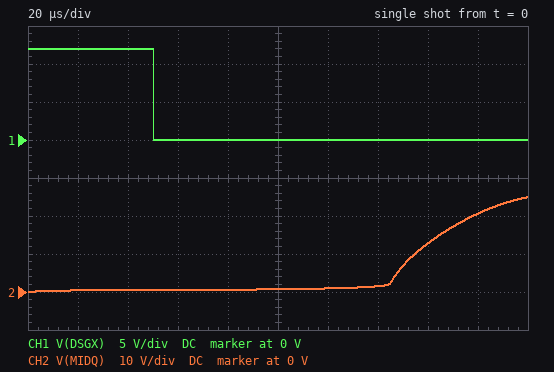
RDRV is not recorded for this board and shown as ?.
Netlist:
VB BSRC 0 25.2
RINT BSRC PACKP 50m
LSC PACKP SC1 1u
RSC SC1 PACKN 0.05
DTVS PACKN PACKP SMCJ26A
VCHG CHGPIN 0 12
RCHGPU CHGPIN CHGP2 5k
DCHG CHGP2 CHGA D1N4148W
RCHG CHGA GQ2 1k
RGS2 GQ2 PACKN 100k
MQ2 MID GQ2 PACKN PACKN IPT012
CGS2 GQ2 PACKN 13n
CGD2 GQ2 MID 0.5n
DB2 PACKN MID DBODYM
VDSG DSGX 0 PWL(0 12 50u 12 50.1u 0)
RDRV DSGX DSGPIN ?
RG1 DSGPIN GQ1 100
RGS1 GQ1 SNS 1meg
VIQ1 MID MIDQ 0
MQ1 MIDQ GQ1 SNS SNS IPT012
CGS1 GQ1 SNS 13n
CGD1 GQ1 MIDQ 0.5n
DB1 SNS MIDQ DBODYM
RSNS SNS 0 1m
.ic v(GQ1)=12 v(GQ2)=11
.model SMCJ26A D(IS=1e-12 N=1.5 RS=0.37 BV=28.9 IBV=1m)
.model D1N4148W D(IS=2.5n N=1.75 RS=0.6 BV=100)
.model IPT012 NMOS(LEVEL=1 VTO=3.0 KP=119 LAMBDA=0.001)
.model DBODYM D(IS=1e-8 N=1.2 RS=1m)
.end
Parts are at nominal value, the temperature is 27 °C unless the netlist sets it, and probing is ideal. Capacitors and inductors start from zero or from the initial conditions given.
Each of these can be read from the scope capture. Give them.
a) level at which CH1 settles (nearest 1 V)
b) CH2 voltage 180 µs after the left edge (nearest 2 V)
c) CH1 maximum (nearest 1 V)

0 V
20 V
12 V
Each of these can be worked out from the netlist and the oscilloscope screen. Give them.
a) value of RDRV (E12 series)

8.2 kΩ
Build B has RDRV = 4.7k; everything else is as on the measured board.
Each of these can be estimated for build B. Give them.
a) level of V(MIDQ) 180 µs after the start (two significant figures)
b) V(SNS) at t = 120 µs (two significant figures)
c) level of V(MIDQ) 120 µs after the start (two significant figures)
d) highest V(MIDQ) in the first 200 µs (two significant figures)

25 V
130 mV
20 V
27 V
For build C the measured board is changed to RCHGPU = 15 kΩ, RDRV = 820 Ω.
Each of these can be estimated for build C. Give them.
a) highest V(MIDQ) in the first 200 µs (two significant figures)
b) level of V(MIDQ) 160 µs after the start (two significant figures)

45 V
25 V
